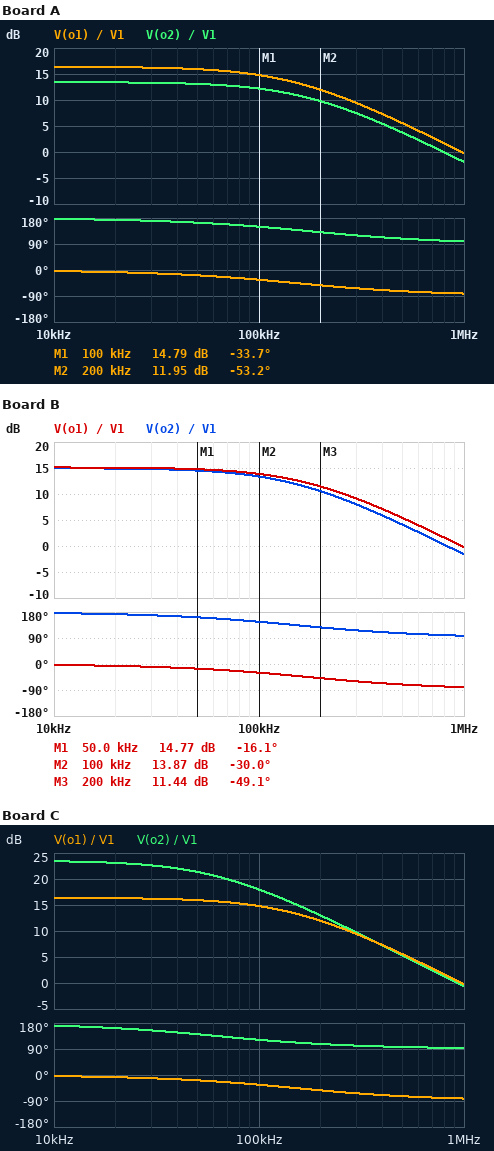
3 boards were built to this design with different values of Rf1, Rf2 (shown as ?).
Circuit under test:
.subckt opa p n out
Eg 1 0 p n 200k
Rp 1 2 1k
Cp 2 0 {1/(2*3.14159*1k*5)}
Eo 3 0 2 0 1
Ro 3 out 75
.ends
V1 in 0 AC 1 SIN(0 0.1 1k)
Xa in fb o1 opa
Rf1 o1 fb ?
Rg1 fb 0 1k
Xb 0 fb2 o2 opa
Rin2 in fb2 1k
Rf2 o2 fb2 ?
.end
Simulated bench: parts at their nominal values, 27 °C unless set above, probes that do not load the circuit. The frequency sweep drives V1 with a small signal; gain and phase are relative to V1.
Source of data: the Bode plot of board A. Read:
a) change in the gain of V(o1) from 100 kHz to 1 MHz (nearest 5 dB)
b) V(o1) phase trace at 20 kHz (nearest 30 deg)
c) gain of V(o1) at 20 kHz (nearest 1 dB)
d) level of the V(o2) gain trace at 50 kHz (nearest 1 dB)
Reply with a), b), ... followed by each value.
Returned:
a) -15 dB
b) 0 deg
c) 16 dB
d) 13 dB
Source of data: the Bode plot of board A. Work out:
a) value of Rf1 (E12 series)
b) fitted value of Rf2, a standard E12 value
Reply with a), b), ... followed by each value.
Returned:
a) 5.6 kΩ
b) 4.7 kΩ
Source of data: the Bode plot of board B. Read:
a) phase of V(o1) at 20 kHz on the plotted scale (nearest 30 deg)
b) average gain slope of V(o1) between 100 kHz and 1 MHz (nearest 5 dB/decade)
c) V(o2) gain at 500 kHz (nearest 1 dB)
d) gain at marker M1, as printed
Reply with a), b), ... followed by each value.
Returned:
a) 0 deg
b) -15 dB/decade
c) 4 dB
d) 14.77 dB
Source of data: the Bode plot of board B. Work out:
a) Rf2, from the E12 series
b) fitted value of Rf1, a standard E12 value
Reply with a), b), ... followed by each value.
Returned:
a) 5.6 kΩ
b) 4.7 kΩ
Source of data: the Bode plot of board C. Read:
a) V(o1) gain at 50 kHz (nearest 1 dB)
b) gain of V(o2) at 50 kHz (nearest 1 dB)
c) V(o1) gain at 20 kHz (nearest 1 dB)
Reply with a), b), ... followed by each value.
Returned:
a) 16 dB
b) 21 dB
c) 16 dB
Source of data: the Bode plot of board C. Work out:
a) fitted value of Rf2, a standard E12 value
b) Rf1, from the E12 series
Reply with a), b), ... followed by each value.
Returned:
a) 15 kΩ
b) 5.6 kΩ
